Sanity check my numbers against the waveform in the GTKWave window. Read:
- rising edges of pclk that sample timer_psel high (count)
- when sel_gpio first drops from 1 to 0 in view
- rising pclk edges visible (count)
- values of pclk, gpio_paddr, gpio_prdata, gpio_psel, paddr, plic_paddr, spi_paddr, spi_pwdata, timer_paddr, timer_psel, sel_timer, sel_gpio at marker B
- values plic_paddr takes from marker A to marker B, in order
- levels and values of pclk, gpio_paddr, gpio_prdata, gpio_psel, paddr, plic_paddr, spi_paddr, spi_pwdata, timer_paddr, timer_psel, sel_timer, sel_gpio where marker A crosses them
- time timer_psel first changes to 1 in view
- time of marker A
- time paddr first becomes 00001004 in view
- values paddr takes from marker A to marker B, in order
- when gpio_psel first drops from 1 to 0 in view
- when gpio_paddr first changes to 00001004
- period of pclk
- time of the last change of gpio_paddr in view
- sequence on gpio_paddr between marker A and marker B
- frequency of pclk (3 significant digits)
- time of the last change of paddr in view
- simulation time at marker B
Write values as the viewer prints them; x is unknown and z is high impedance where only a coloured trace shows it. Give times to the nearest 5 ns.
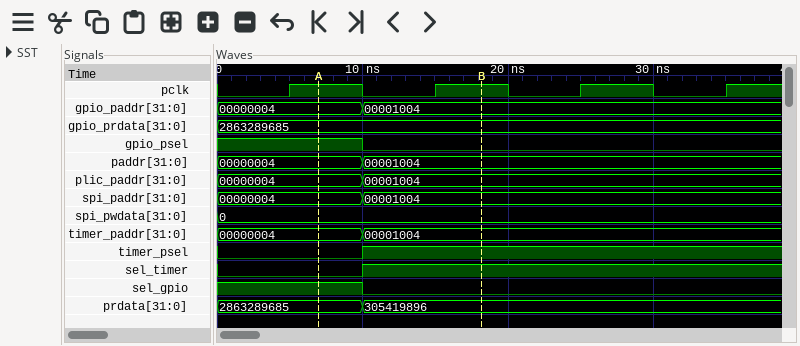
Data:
3
10 ns
4
pclk=1, gpio_paddr=00001004, gpio_prdata=2863289685, gpio_psel=0, paddr=00001004, plic_paddr=00001004, spi_paddr=00001004, spi_pwdata=0, timer_paddr=00001004, timer_psel=1, sel_timer=1, sel_gpio=0
00000004, 00001004
pclk=1, gpio_paddr=00000004, gpio_prdata=2863289685, gpio_psel=1, paddr=00000004, plic_paddr=00000004, spi_paddr=00000004, spi_pwdata=0, timer_paddr=00000004, timer_psel=0, sel_timer=0, sel_gpio=1
10 ns
5 ns
10 ns
00000004, 00001004
10 ns
10 ns
10 ns
10 ns
00000004, 00001004
100 MHz
10 ns
20 ns
